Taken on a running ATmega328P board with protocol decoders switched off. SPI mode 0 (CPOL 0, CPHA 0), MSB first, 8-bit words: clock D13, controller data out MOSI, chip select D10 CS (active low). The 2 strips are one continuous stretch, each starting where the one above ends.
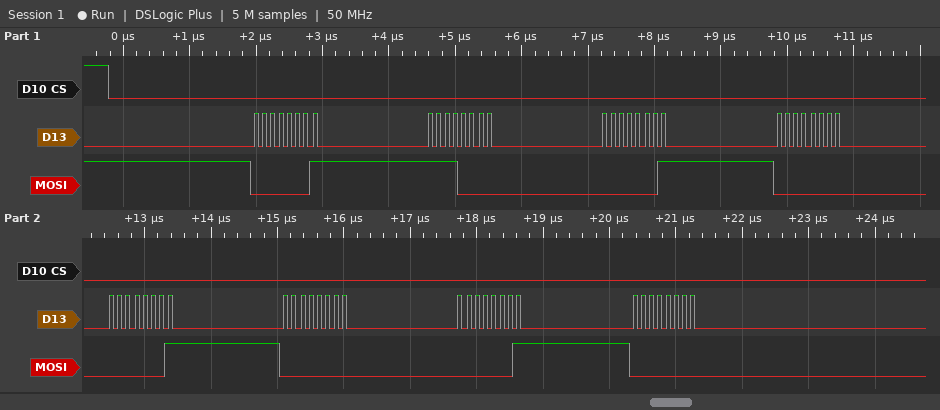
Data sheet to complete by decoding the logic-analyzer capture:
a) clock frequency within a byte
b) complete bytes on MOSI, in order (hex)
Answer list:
8 MHz
01 F0 01 00 01 00 01 00
